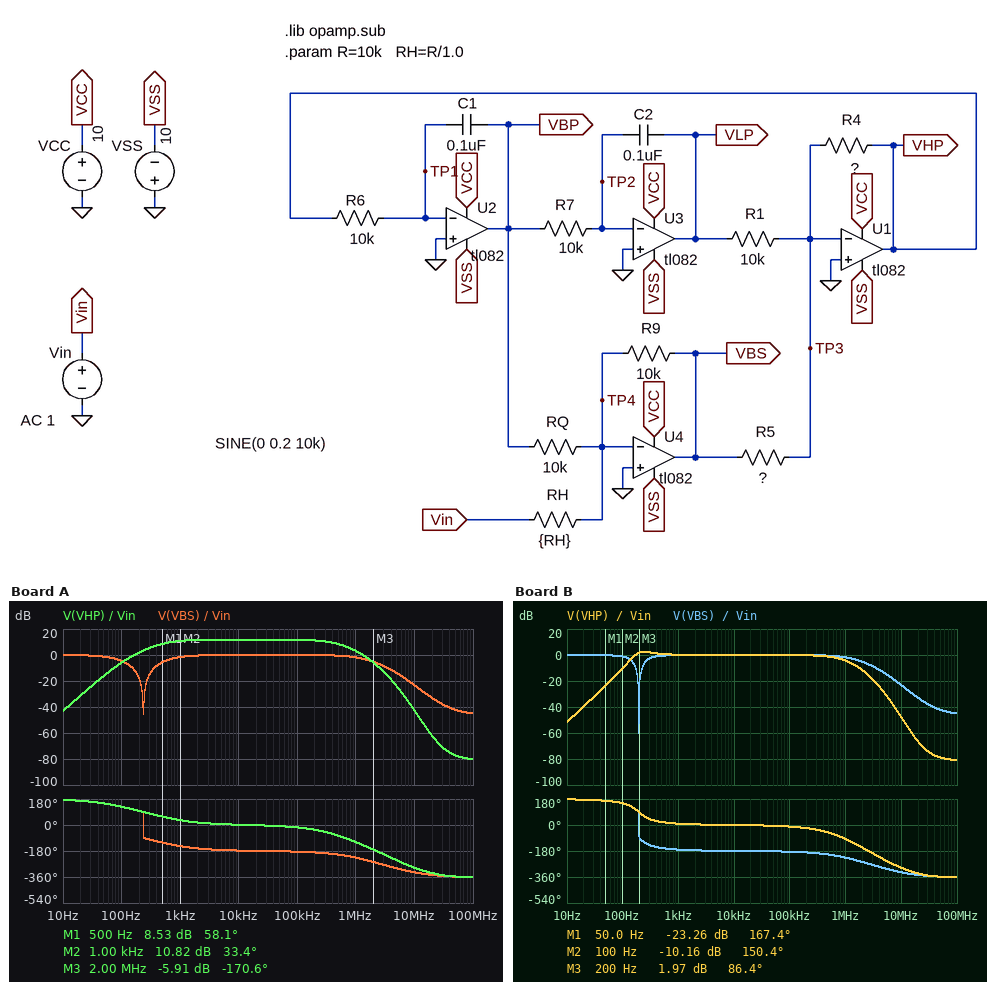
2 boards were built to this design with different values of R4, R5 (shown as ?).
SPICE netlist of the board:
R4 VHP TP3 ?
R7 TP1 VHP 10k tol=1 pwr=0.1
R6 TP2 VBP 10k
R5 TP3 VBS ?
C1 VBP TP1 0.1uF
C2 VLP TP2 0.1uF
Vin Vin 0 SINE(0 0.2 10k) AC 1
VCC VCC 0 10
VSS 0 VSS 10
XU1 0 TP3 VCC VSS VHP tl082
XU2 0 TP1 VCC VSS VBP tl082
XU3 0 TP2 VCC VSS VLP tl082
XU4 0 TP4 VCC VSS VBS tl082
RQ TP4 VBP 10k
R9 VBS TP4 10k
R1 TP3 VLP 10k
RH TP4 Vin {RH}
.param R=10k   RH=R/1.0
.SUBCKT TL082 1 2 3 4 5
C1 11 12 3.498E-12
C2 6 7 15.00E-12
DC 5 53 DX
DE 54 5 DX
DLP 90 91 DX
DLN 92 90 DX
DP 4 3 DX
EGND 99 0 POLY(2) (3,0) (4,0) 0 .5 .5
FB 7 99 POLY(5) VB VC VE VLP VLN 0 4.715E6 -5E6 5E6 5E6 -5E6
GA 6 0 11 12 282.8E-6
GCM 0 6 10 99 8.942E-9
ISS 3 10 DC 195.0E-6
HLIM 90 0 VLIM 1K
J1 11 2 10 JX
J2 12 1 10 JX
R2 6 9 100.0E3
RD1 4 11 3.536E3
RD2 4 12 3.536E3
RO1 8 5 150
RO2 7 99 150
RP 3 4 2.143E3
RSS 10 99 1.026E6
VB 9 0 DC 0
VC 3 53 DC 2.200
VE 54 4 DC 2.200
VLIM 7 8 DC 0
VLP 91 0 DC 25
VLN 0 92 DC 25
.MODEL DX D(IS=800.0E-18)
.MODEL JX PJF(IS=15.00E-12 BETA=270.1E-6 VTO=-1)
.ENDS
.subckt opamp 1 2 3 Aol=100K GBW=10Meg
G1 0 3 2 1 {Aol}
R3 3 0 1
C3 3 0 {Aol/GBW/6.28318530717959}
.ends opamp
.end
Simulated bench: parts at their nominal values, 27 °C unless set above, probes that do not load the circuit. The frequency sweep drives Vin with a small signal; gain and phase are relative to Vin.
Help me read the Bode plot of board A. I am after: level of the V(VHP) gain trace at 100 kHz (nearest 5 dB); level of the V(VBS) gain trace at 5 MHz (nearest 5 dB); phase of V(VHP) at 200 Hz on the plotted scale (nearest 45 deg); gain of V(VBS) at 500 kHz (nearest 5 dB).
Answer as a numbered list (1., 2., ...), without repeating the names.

1. 10 dB
2. -15 dB
3. 90 deg
4. 0 dB
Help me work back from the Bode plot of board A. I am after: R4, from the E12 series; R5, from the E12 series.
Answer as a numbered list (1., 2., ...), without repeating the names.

1. 22 kΩ
2. 5.6 kΩ
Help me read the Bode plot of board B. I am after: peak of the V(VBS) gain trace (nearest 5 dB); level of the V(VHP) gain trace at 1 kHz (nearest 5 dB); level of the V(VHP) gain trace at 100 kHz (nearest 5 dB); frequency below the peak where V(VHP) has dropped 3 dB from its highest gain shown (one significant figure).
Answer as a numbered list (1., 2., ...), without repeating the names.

1. 0 dB
2. 0 dB
3. 0 dB
4. 200 Hz
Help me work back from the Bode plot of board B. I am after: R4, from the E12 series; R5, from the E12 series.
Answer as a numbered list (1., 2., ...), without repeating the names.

1. 15 kΩ
2. 15 kΩ
